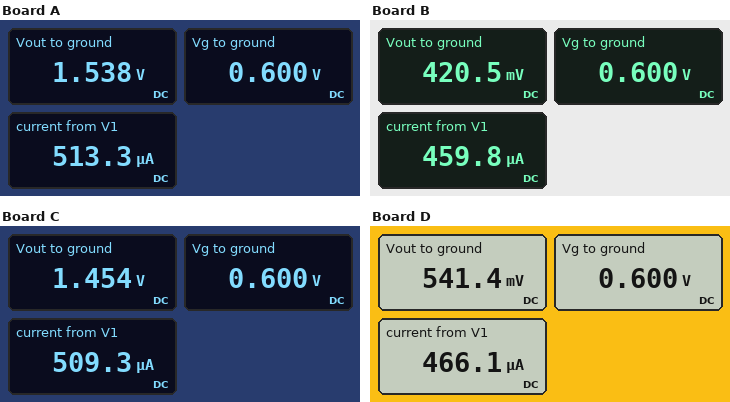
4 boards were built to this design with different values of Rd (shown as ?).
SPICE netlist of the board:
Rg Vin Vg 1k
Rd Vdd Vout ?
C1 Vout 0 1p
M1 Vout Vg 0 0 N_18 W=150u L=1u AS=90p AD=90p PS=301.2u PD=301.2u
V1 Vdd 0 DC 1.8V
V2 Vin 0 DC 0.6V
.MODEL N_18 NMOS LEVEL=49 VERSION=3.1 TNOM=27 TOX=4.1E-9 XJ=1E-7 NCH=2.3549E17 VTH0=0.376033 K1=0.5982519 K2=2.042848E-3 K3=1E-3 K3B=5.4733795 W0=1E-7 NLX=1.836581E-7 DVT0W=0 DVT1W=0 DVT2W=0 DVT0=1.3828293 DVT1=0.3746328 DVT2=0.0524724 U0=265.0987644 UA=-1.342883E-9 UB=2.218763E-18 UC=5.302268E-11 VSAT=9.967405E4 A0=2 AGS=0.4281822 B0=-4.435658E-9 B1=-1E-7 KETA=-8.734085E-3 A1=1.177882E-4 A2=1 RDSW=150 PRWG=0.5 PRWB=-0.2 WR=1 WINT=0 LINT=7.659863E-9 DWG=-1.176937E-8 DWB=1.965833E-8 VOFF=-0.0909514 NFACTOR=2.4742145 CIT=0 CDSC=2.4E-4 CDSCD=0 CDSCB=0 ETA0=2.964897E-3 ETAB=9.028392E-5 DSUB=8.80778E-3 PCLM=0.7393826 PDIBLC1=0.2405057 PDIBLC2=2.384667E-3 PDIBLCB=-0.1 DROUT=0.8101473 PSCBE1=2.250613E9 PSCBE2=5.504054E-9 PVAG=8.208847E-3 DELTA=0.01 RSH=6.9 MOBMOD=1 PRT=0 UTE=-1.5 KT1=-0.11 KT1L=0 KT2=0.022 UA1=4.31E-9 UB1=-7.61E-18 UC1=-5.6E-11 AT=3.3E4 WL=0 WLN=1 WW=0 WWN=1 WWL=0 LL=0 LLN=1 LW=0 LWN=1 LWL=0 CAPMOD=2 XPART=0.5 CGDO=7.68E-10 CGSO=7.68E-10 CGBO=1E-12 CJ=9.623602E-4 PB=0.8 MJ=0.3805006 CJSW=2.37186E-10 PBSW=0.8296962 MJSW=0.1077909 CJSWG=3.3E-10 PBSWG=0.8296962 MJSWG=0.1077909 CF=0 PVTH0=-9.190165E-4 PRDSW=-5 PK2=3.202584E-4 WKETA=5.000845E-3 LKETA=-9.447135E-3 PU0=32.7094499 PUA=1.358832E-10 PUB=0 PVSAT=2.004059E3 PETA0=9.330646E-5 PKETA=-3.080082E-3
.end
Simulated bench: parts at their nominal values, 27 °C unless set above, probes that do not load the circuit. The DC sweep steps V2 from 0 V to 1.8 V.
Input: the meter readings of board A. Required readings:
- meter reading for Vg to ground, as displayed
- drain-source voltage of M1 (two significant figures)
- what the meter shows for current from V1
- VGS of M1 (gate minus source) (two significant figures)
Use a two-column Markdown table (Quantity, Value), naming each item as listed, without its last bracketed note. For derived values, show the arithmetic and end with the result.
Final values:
| Quantity | Value |
|---|---|
| meter reading for Vg to ground, as displayed | 0.600 V |
| drain-source voltage of M1 | 1.538 V = 1.5 V |
| what the meter shows for current from V1 | 513.3 µA |
| VGS of M1 (gate minus source) | 600 mV = 600 mV |
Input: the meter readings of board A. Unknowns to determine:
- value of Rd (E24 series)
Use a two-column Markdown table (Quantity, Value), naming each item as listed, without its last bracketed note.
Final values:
| Quantity | Value |
|---|---|
| value of Rd | 510 Ω |
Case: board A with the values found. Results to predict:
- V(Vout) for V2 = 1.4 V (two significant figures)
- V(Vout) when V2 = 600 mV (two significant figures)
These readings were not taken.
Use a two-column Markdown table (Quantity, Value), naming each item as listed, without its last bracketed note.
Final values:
| Quantity | Value |
|---|---|
| V(Vout) for V2 = 1.4 V | 140 mV |
| V(Vout) when V2 = 600 mV | 1.5 V |
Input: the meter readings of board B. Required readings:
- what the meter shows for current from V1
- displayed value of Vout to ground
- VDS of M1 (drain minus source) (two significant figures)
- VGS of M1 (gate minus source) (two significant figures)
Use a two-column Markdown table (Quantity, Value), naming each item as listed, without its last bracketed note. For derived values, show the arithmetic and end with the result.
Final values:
| Quantity | Value |
|---|---|
| what the meter shows for current from V1 | 459.8 µA |
| displayed value of Vout to ground | 420.5 mV |
| VDS of M1 (drain minus source) | 420.5 mV = 420 mV |
| VGS of M1 (gate minus source) | 600 mV = 600 mV |
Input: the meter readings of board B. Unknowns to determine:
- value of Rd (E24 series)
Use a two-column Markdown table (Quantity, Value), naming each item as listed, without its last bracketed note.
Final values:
| Quantity | Value |
|---|---|
| value of Rd | 3 kΩ |
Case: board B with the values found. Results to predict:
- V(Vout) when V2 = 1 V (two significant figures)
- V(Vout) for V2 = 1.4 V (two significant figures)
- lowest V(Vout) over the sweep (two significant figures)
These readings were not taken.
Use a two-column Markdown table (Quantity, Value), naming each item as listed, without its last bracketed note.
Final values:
| Quantity | Value |
|---|---|
| V(Vout) when V2 = 1 V | 35 mV |
| V(Vout) for V2 = 1.4 V | 25 mV |
| lowest V(Vout) over the sweep | 21 mV |
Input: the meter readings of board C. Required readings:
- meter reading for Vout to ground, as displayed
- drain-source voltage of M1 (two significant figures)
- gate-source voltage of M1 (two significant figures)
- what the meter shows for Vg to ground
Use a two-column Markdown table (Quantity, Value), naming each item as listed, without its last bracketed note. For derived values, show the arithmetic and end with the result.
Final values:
| Quantity | Value |
|---|---|
| meter reading for Vout to ground, as displayed | 1.454 V |
| drain-source voltage of M1 | 1.454 V = 1.5 V |
| gate-source voltage of M1 | 600 mV = 600 mV |
| what the meter shows for Vg to ground | 0.600 V |
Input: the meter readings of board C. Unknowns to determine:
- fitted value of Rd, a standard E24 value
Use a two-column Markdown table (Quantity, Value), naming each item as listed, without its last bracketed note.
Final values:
| Quantity | Value |
|---|---|
| fitted value of Rd, a standard E24 value | 680 Ω |
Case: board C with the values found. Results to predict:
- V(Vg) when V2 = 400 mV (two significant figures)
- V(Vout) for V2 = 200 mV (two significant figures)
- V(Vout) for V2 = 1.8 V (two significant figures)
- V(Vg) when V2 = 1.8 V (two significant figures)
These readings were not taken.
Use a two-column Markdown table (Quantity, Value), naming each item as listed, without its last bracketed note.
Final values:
| Quantity | Value |
|---|---|
| V(Vg) when V2 = 400 mV | 400 mV |
| V(Vout) for V2 = 200 mV | 1.8 V |
| V(Vout) for V2 = 1.8 V | 92 mV |
| V(Vg) when V2 = 1.8 V | 1.8 V |
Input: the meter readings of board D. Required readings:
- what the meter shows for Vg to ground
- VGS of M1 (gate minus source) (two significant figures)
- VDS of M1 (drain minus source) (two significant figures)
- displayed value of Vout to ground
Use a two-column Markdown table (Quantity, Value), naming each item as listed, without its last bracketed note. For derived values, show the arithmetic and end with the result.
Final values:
| Quantity | Value |
|---|---|
| what the meter shows for Vg to ground | 0.600 V |
| VGS of M1 (gate minus source) | 600 mV = 600 mV |
| VDS of M1 (drain minus source) | 541.4 mV = 540 mV |
| displayed value of Vout to ground | 541.4 mV |
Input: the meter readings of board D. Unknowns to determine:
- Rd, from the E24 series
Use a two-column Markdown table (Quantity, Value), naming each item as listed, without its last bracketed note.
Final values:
| Quantity | Value |
|---|---|
| Rd, from the E24 series | 2.7 kΩ |
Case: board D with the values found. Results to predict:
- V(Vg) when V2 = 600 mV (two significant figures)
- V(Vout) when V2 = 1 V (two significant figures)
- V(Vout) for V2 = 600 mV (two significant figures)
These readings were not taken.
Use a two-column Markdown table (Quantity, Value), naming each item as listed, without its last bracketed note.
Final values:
| Quantity | Value |
|---|---|
| V(Vg) when V2 = 600 mV | 600 mV |
| V(Vout) when V2 = 1 V | 39 mV |
| V(Vout) for V2 = 600 mV | 540 mV |
